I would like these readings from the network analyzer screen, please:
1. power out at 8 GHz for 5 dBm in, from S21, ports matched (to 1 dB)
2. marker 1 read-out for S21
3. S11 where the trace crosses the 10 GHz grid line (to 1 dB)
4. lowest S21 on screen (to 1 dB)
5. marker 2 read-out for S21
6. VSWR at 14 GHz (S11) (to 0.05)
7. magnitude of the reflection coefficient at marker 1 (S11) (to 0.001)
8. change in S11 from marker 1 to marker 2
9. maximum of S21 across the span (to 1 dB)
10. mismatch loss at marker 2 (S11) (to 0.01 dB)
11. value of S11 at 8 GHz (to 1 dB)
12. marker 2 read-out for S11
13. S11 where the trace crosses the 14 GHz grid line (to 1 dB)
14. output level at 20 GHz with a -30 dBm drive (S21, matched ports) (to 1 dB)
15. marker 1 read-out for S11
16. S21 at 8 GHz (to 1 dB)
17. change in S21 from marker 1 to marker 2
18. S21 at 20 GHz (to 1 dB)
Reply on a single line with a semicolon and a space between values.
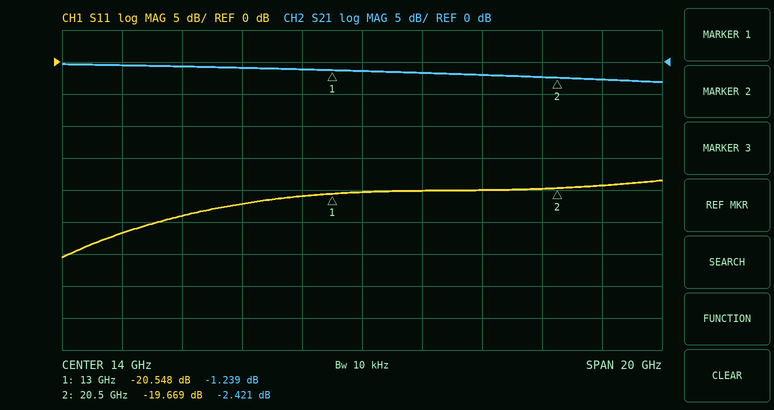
4 dBm; -1.239 dB; -22 dB; -3 dB; -2.421 dB; 1.20; 0.094; 0.879 dB; 0 dB; 0.05 dB; -24 dB; -19.669 dB; -20 dB; -32 dBm; -20.548 dB; -1 dB; -1.182 dB; -2 dB
